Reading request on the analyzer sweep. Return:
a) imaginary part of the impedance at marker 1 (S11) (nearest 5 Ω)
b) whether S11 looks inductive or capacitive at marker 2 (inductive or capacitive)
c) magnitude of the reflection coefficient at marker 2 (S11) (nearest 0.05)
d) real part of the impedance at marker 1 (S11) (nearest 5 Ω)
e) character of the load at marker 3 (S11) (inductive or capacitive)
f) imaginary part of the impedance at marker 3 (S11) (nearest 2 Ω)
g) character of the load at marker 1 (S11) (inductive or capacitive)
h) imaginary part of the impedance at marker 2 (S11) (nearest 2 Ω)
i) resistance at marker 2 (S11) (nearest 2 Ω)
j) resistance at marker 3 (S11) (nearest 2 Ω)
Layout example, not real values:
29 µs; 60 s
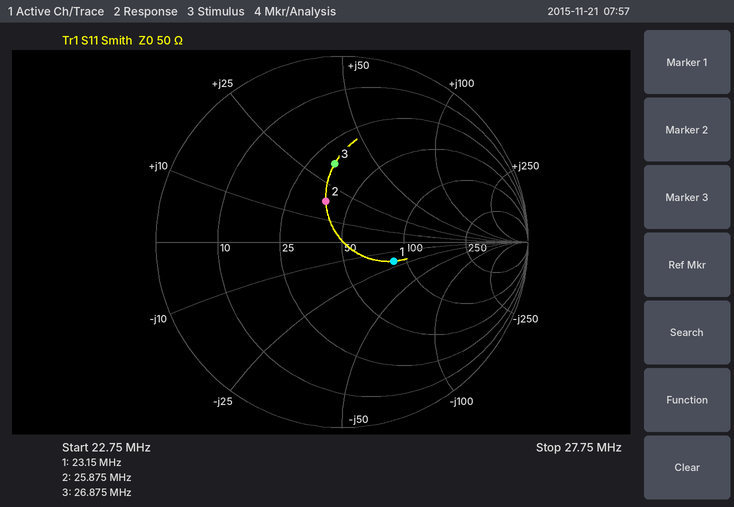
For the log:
-20 Ω; inductive; 0.25; 85 Ω; inductive; +34 Ω; capacitive; +18 Ω; 38 Ω; 32 Ω
